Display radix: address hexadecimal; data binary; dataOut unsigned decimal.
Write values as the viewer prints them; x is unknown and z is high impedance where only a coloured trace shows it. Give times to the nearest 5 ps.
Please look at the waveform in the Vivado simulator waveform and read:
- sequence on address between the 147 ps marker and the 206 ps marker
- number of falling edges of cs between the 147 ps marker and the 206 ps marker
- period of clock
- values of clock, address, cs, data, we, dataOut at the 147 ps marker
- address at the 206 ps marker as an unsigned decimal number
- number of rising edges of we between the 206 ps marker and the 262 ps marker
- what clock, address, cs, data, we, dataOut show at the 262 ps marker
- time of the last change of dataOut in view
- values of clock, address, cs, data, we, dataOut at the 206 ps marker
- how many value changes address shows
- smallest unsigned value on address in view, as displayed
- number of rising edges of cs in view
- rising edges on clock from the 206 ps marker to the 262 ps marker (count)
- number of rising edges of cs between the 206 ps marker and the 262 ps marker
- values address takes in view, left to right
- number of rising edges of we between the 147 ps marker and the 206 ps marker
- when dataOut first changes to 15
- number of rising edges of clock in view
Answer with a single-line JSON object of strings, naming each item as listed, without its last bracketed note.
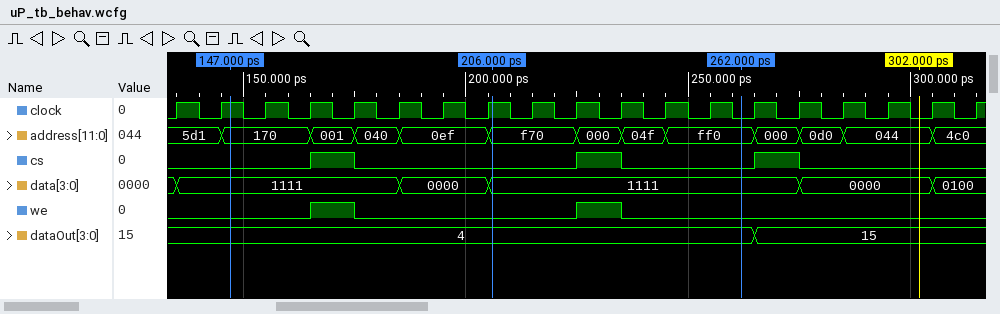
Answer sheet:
{"sequence on address between the 147 ps marker and the 206 ps marker": "170, 001, 040, 0ef, f70", "number of falling edges of cs between the 147 ps marker and the 206 ps marker": "1", "period of clock": "10 ps", "values of clock, address, cs, data, we, dataOut at the 147 ps marker": "clock=1, address=170, cs=0, data=1111, we=0, dataOut=4", "address at the 206 ps marker as an unsigned decimal number": "3952", "number of rising edges of we between the 206 ps marker and the 262 ps marker": "1", "what clock, address, cs, data, we, dataOut show at the 262 ps marker": "clock=0, address=ff0, cs=0, data=1111, we=0, dataOut=4", "time of the last change of dataOut in view": "265 ps", "values of clock, address, cs, data, we, dataOut at the 206 ps marker": "clock=1, address=f70, cs=0, data=1111, we=0, dataOut=4", "how many value changes address shows": "12", "smallest unsigned value on address in view, as displayed": "000", "number of rising edges of cs in view": "3", "rising edges on clock from the 206 ps marker to the 262 ps marker": "5", "number of rising edges of cs between the 206 ps marker and the 262 ps marker": "1", "values address takes in view, left to right": "5d1, 170, 001, 040, 0ef, f70, 000, 04f, ff0, 000, 0d0, 044, 4c0", "number of rising edges of we between the 147 ps marker and the 206 ps marker": "1", "when dataOut first changes to 15": "265 ps", "number of rising edges of clock in view": "19"}
